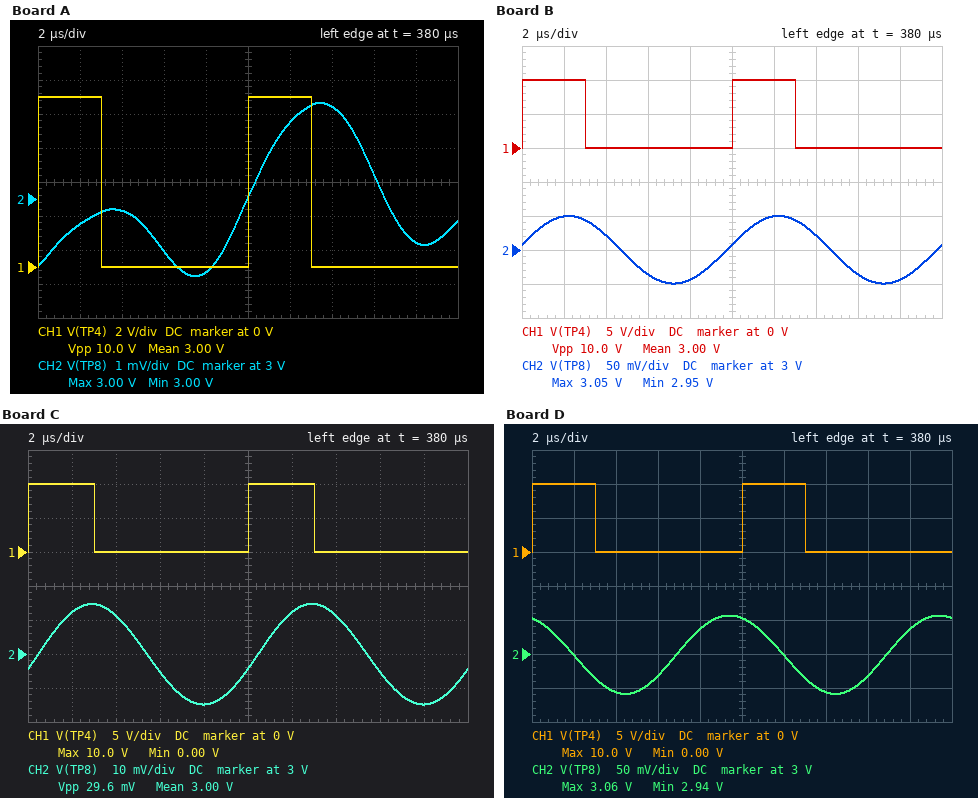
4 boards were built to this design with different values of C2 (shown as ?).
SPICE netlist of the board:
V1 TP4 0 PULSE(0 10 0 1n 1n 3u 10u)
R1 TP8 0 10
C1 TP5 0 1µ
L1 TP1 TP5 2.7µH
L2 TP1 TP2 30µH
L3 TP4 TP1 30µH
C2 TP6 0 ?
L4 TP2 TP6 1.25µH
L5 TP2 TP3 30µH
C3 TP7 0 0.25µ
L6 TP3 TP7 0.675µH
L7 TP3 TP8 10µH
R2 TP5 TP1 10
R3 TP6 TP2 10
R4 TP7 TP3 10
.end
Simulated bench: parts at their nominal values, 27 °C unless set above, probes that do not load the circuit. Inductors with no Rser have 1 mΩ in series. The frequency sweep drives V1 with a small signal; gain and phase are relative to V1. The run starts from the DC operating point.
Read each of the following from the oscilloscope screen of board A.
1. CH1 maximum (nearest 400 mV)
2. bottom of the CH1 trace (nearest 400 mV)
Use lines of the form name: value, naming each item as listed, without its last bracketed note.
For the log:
CH1 maximum: 10.0 V
bottom of the CH1 trace: 0 V
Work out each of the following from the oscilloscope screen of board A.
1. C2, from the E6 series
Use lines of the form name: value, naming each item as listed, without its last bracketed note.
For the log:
C2, from the E6 series: 1 µF
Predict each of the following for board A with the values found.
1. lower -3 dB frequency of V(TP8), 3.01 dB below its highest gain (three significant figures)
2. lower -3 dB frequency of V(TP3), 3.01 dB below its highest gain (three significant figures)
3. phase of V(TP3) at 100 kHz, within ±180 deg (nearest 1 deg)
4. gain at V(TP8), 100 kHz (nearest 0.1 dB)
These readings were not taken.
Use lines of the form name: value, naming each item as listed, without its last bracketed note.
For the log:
lower -3 dB frequency of V(TP8), 3.01 dB below its highest gain: 10.1 kHz
lower -3 dB frequency of V(TP3), 3.01 dB below its highest gain: 10.2 kHz
phase of V(TP3) at 100 kHz, within ±180 deg: -25 deg
gain at V(TP8), 100 kHz: -69.8 dB
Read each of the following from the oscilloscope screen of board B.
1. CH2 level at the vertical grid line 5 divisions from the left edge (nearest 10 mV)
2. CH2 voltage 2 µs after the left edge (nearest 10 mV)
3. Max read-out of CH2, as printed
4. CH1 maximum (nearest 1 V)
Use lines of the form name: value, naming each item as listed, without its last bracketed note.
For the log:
CH2 level at the vertical grid line 5 divisions from the left edge: 3.01 V
CH2 voltage 2 µs after the left edge: 3.05 V
Max read-out of CH2, as printed: 3.05 V
CH1 maximum: 10 V
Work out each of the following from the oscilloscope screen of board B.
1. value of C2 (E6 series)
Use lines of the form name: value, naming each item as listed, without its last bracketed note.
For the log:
value of C2: 220 nF
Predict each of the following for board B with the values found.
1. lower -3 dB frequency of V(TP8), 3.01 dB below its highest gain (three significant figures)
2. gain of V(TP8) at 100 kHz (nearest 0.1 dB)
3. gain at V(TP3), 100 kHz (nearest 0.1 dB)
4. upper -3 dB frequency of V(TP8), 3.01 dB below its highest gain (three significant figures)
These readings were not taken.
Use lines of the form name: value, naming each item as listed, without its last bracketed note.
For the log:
lower -3 dB frequency of V(TP8), 3.01 dB below its highest gain: 19.7 kHz
gain of V(TP8) at 100 kHz: -40.3 dB
gain at V(TP3), 100 kHz: -38.9 dB
upper -3 dB frequency of V(TP8), 3.01 dB below its highest gain: 34.7 kHz
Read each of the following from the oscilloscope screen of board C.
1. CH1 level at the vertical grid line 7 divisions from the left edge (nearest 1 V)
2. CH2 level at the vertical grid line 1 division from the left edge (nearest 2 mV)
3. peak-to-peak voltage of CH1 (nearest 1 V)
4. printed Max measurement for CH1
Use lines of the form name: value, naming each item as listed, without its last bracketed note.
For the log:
CH1 level at the vertical grid line 7 divisions from the left edge: 0 V
CH2 level at the vertical grid line 1 division from the left edge: 3.012 V
peak-to-peak voltage of CH1: 10 V
printed Max measurement for CH1: 10.0 V
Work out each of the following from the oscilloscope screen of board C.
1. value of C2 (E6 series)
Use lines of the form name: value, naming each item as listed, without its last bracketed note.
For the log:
value of C2: 330 nF
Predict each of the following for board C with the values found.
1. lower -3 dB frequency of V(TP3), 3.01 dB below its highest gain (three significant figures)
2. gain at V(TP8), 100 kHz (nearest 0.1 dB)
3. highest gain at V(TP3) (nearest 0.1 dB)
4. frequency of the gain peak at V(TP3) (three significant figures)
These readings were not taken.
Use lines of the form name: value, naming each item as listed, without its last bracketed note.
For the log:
lower -3 dB frequency of V(TP3), 3.01 dB below its highest gain: 16.6 kHz
gain at V(TP8), 100 kHz: -50.8 dB
highest gain at V(TP3): 5.3 dB
frequency of the gain peak at V(TP3): 27.4 kHz
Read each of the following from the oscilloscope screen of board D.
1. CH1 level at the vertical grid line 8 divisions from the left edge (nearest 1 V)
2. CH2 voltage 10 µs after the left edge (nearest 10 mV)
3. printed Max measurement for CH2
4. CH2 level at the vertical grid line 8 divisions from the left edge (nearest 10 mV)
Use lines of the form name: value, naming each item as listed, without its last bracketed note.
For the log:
CH1 level at the vertical grid line 8 divisions from the left edge: 0 V
CH2 voltage 10 µs after the left edge: 3.05 V
printed Max measurement for CH2: 3.06 V
CH2 level at the vertical grid line 8 divisions from the left edge: 2.97 V
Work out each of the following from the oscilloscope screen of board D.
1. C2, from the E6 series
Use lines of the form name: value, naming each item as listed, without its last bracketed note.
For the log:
C2, from the E6 series: 150 nF
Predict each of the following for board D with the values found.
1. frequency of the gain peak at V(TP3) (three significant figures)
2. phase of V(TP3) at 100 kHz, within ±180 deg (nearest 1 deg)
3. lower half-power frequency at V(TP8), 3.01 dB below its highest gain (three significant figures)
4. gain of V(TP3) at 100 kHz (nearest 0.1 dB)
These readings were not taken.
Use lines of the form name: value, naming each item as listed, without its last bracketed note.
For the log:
frequency of the gain peak at V(TP3): 29.8 kHz
phase of V(TP3) at 100 kHz, within ±180 deg: 107 deg
lower half-power frequency at V(TP8), 3.01 dB below its highest gain: 21.8 kHz
gain of V(TP3) at 100 kHz: -37.6 dB
